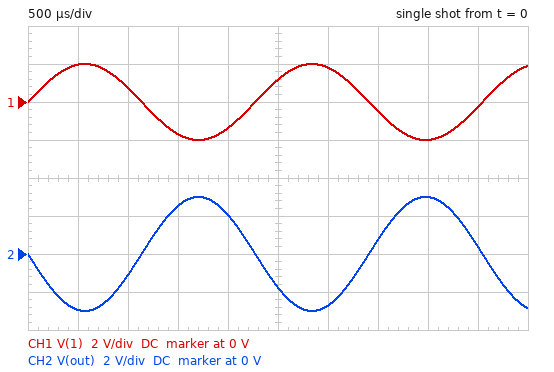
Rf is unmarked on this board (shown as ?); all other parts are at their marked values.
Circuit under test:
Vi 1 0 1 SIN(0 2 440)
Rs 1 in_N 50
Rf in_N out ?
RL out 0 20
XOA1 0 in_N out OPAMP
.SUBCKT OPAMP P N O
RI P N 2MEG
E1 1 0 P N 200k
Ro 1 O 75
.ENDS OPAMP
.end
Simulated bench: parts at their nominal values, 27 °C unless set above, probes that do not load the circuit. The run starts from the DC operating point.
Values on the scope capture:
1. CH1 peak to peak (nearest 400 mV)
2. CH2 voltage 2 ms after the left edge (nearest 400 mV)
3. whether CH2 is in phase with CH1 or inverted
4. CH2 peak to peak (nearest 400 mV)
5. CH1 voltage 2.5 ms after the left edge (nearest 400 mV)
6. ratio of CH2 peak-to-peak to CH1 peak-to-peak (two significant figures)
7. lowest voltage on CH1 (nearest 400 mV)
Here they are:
4.0 V
2.0 V
inverted
6.0 V
1.2 V
1.5
-2.0 V
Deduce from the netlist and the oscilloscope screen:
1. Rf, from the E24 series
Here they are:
75 Ω
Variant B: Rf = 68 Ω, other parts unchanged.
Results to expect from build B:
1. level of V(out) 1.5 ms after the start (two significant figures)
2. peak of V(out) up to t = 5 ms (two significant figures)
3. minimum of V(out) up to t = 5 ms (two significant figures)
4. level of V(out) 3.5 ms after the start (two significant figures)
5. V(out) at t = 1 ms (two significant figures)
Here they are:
2.3 V
2.7 V
-2.7 V
680 mV
-1.0 V
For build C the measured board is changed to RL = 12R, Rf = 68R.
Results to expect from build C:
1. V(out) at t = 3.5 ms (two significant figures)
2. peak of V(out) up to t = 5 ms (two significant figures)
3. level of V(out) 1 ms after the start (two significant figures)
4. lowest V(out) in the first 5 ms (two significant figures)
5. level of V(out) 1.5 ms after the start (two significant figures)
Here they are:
680 mV
2.7 V
-1.0 V
-2.7 V
2.3 V
